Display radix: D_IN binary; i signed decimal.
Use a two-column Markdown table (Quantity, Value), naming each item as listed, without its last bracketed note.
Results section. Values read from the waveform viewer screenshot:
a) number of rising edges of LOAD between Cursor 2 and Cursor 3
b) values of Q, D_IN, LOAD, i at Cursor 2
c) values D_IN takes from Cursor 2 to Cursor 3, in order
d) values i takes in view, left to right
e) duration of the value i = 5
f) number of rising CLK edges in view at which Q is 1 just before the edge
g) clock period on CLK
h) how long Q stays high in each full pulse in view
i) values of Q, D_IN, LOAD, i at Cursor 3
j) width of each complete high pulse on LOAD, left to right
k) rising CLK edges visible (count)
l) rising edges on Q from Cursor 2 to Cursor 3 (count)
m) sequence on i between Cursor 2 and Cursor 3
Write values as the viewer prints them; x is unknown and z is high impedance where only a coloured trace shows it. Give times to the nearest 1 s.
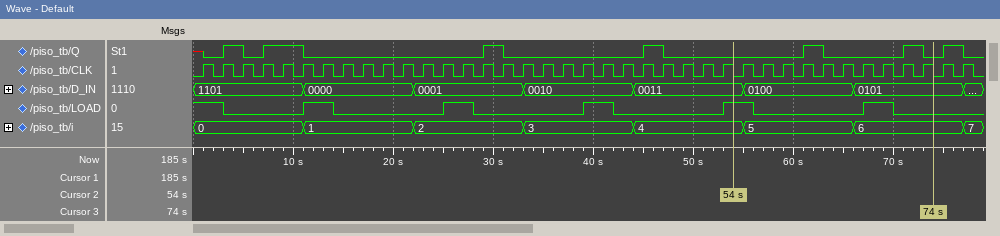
| Quantity | Value |
|---|---|
| number of rising edges of LOAD between Cursor 2 and Cursor 3 | 1 |
| values of Q, D_IN, LOAD, i at Cursor 2 | Q=0, D_IN=0011, LOAD=1, i=4 |
| values D_IN takes from Cursor 2 to Cursor 3, in order | 0011, 0100, 0101 |
| values i takes in view, left to right | 0, 1, 2, 3, 4, 5, 6, 7 |
| duration of the value i = 5 | 11 s |
| number of rising CLK edges in view at which Q is 1 just before the edge | 8 |
| clock period on CLK | 2 s |
| how long Q stays high in each full pulse in view | 2 s, 4 s, 2 s, 2 s, 2 s, 2 s, 2 s |
| values of Q, D_IN, LOAD, i at Cursor 3 | Q=0, D_IN=0101, LOAD=0, i=6 |
| width of each complete high pulse on LOAD, left to right | 3 s, 3 s, 3 s, 3 s, 3 s |
| rising CLK edges visible | 39 |
| rising edges on Q from Cursor 2 to Cursor 3 | 2 |
| sequence on i between Cursor 2 and Cursor 3 | 4, 5, 6 |
